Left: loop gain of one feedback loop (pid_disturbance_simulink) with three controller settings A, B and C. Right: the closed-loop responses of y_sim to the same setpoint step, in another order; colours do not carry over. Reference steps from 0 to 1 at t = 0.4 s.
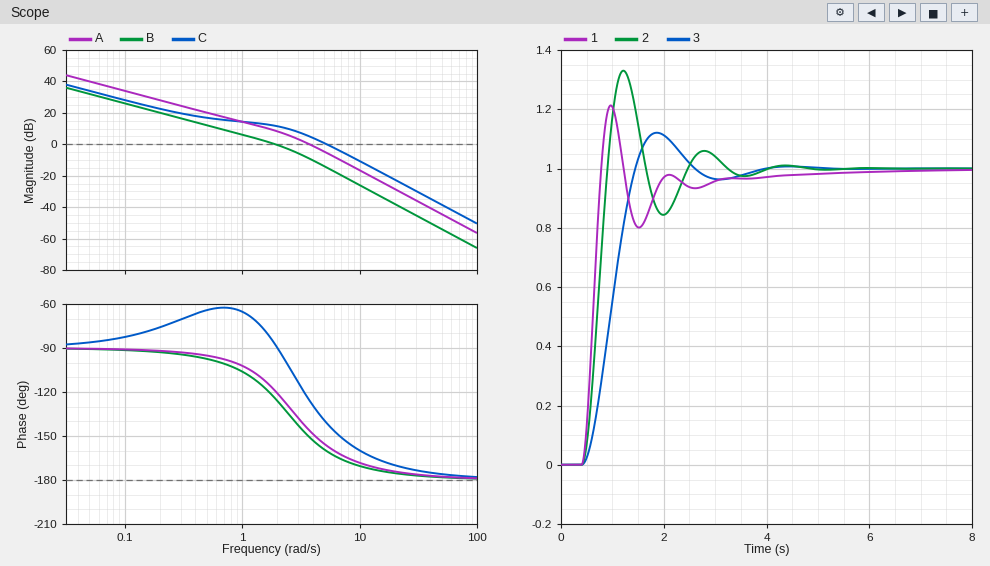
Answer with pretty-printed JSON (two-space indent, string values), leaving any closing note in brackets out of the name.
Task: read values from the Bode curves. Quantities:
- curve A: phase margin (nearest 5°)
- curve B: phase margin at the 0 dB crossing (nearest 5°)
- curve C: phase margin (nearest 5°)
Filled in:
{
  "curve A: phase margin": "35°",
  "curve B: phase margin at the 0 dB crossing": "55°",
  "curve C: phase margin": "40°"
}
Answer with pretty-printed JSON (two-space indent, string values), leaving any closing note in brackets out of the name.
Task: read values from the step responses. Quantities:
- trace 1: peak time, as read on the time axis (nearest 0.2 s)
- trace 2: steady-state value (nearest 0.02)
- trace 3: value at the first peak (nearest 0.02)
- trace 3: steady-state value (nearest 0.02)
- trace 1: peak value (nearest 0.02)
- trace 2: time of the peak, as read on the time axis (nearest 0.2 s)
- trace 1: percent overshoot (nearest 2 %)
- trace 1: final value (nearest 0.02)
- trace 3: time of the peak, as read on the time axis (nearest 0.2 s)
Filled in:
{
  "trace 1: peak time, as read on the time axis": "1.0 s",
  "trace 2: steady-state value": "1.00",
  "trace 3: value at the first peak": "1.12",
  "trace 3: steady-state value": "1.00",
  "trace 1: peak value": "1.22",
  "trace 2: time of the peak, as read on the time axis": "1.2 s",
  "trace 1: percent overshoot": "22 %",
  "trace 1: final value": "1.00",
  "trace 3: time of the peak, as read on the time axis": "1.8 s"
}
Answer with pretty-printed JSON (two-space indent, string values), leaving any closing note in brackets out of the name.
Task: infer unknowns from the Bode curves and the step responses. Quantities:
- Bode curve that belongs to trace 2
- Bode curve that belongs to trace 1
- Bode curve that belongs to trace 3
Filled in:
{
  "Bode curve that belongs to trace 2": "A",
  "Bode curve that belongs to trace 1": "C",
  "Bode curve that belongs to trace 3": "B"
}
